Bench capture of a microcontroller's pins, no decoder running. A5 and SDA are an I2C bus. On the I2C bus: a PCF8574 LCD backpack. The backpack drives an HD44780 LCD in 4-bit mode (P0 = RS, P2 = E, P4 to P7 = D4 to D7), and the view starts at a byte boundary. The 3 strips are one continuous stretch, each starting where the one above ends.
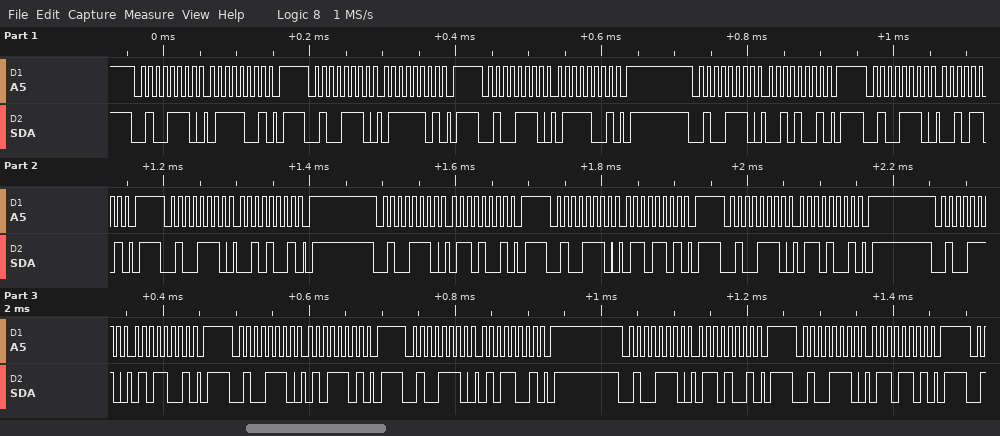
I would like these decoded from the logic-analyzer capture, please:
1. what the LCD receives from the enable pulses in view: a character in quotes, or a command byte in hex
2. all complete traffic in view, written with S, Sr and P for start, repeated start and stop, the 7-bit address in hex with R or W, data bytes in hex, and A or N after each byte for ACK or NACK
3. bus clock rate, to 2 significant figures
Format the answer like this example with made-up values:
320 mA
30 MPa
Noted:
'r' 'e'
S 27W A 79 A P S 27W A 7D A P S 27W A 79 A P S 27W A 29 A P S 27W A 2D A P S 27W A 29 A P S 27W A 69 A P S 27W A 6D A P S 27W A 69 A P S 27W A 59 A P S 27W A 5D A P S 27W A 59 A P S 27W A 69 A P S 27W A 6D A P
100 kHz
